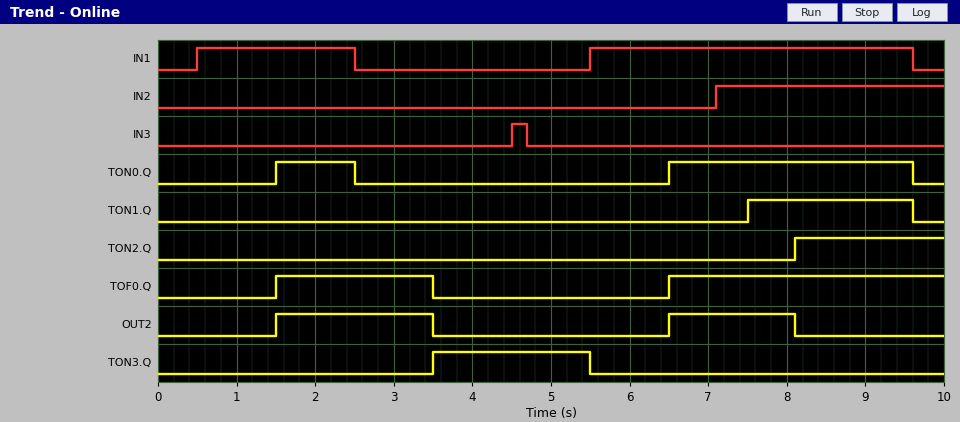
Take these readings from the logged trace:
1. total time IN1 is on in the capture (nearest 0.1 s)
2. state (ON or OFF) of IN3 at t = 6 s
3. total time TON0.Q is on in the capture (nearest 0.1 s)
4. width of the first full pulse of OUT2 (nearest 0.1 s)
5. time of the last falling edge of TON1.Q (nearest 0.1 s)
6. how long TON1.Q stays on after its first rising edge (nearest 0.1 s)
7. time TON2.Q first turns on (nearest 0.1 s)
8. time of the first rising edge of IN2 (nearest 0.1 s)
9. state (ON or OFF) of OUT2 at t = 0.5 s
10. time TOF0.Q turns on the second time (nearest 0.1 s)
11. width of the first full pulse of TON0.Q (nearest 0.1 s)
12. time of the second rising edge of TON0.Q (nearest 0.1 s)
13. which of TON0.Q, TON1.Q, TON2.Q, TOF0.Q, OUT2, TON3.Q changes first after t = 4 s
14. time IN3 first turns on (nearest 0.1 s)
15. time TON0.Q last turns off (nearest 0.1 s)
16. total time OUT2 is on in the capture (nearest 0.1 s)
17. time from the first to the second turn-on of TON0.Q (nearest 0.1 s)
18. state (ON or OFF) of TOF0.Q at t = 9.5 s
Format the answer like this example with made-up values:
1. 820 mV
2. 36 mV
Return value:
1. 6.1 s
2. OFF
3. 4.1 s
4. 2.0 s
5. 9.6 s
6. 2.1 s
7. 8.1 s
8. 7.1 s
9. OFF
10. 6.5 s
11. 1.0 s
12. 6.5 s
13. TON3.Q
14. 4.5 s
15. 9.6 s
16. 3.6 s
17. 5.0 s
18. ON
